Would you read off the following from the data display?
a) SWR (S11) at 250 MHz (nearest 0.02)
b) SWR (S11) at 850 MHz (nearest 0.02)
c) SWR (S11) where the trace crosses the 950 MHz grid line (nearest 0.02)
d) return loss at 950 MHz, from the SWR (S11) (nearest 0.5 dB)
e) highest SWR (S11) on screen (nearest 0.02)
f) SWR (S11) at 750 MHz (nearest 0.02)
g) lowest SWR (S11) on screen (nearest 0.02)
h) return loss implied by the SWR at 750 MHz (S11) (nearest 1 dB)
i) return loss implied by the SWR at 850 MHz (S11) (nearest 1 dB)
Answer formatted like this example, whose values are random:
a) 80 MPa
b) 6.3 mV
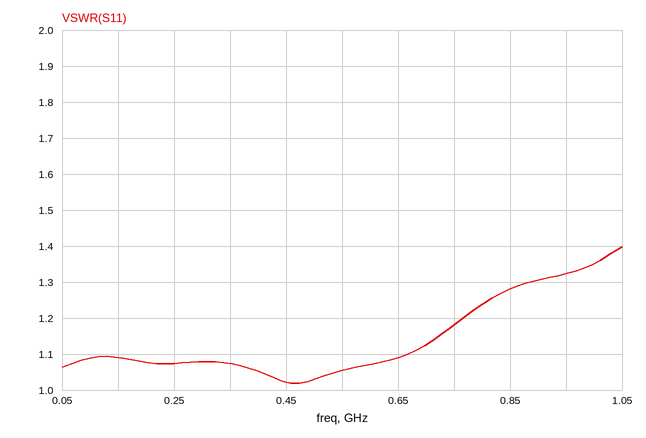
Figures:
a) 1.08
b) 1.28
c) 1.32
d) 17.0 dB
e) 1.40
f) 1.18
g) 1.02
h) 22 dB
i) 18 dB
